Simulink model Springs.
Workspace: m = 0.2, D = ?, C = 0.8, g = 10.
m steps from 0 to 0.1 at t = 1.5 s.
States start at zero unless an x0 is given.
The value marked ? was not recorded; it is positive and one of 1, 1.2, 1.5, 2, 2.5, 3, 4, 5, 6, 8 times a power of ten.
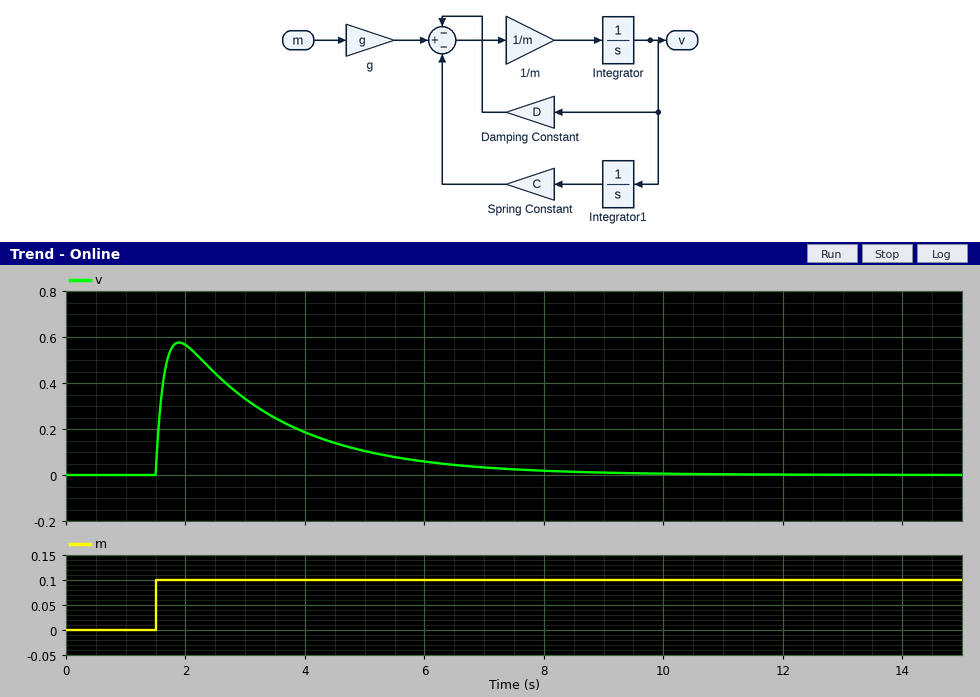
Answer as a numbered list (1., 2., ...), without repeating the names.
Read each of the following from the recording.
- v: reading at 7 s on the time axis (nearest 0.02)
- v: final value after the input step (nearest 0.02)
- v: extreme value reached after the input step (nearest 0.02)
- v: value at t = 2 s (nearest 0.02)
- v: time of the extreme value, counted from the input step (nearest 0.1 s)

1. 0.04
2. 0.00
3. 0.58
4. 0.56
5. 0.4 s
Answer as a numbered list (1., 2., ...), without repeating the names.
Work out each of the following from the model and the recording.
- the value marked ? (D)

1. 1.5
